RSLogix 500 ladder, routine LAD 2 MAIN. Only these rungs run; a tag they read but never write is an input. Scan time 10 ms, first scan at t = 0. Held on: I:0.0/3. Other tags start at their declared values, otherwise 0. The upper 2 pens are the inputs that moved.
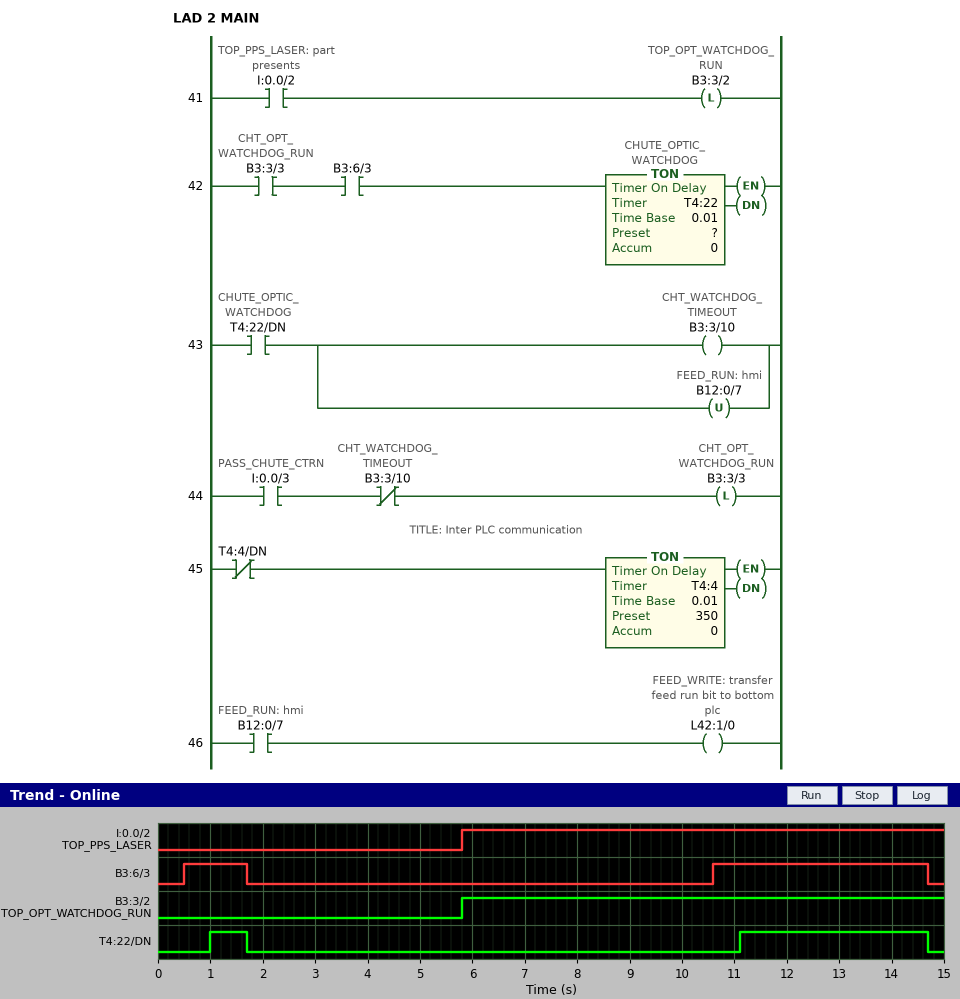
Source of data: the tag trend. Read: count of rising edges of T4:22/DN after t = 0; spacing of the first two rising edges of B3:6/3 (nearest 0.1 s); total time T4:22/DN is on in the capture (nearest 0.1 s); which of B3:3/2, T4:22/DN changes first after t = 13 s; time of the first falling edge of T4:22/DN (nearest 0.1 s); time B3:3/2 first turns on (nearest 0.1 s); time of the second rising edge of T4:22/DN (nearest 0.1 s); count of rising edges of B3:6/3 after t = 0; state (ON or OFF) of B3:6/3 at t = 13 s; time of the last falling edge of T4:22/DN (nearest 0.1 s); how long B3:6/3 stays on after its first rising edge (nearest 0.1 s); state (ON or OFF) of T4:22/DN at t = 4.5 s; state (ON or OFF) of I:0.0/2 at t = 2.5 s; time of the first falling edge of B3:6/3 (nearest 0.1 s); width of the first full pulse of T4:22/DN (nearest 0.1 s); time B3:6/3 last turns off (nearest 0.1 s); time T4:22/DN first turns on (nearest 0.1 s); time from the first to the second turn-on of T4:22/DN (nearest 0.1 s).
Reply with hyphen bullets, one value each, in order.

- 2
- 10.1 s
- 4.3 s
- T4:22/DN
- 1.7 s
- 5.8 s
- 11.1 s
- 2
- ON
- 14.7 s
- 1.2 s
- OFF
- OFF
- 1.7 s
- 0.7 s
- 14.7 s
- 1.0 s
- 10.1 s
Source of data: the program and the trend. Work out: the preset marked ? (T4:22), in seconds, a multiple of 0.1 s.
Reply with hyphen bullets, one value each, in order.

- 0.5 s
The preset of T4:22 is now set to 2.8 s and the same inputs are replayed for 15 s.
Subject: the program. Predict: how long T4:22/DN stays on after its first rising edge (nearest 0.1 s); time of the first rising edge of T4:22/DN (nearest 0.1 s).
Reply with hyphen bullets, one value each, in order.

- 1.3 s
- 13.4 s
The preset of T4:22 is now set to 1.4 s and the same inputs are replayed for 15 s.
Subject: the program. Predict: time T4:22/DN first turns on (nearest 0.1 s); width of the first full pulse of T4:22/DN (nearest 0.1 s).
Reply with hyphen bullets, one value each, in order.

- 12.0 s
- 2.7 s
